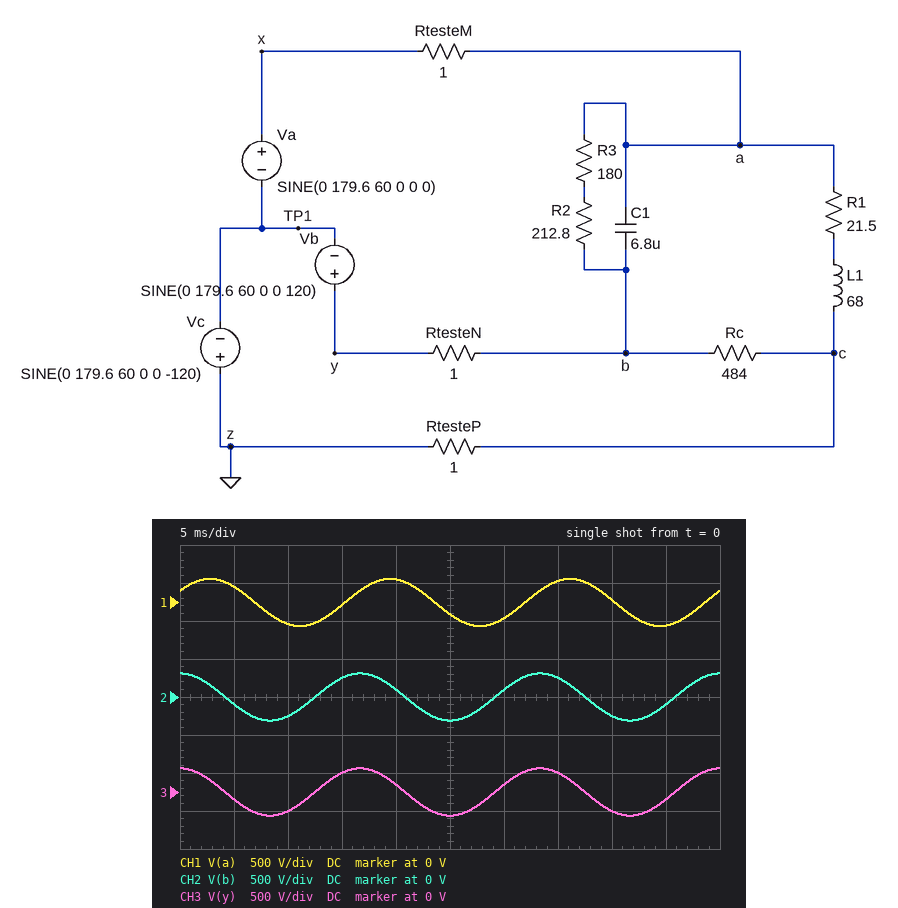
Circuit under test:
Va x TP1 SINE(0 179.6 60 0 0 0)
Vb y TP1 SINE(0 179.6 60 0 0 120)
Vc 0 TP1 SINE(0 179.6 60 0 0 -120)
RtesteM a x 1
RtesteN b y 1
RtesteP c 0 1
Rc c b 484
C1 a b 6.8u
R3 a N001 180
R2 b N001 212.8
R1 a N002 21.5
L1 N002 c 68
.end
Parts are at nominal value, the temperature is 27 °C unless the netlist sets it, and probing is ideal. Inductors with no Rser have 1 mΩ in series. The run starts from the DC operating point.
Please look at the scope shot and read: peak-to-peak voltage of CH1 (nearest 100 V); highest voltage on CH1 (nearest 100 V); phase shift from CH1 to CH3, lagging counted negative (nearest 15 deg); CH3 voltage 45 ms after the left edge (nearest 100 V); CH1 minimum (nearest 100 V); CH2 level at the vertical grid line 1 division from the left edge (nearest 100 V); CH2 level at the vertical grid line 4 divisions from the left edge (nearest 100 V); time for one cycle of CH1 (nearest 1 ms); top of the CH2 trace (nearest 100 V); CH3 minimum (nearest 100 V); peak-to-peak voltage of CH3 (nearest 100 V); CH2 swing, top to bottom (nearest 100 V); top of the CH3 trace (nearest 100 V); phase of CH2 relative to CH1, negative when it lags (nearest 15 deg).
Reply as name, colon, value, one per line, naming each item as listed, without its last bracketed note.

peak-to-peak voltage of CH1: 600 V
highest voltage on CH1: 300 V
phase shift from CH1 to CH3, lagging counted negative: 60 deg
CH3 voltage 45 ms after the left edge: -100 V
CH1 minimum: -300 V
CH2 level at the vertical grid line 1 division from the left edge: -100 V
CH2 level at the vertical grid line 4 divisions from the left edge: 100 V
time for one cycle of CH1: 17 ms
top of the CH2 trace: 300 V
CH3 minimum: -300 V
peak-to-peak voltage of CH3: 600 V
CH2 swing, top to bottom: 600 V
top of the CH3 trace: 300 V
phase of CH2 relative to CH1, negative when it lags: 60 deg
